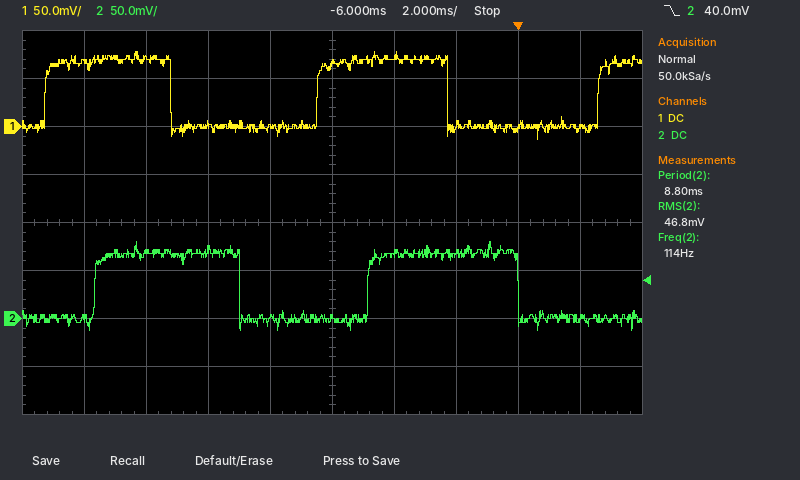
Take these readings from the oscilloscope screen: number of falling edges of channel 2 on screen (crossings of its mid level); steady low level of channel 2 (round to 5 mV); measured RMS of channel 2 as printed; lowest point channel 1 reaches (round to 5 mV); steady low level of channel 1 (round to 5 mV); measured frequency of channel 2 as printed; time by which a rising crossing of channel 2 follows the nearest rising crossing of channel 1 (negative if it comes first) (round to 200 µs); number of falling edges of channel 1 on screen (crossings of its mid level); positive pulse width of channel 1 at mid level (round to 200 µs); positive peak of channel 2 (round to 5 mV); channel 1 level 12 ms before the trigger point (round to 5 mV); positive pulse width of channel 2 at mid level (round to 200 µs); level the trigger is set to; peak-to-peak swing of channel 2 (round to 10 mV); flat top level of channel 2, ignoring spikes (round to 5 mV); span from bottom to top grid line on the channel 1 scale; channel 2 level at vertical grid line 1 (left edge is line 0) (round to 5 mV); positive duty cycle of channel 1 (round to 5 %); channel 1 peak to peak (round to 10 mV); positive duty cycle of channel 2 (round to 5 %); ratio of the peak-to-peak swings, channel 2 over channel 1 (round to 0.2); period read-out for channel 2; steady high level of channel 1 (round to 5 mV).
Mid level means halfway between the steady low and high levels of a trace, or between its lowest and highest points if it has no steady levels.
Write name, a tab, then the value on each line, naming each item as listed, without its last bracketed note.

number of falling edges of channel 2 on screen	2
steady low level of channel 2	0 mV
measured RMS of channel 2 as printed	46.8 mV
lowest point channel 1 reaches	-15 mV
steady low level of channel 1	0 mV
measured frequency of channel 2 as printed	114 Hz
time by which a rising crossing of channel 2 follows the nearest rising crossing of channel 1 (negative if it comes first)	+1.6 ms
number of falling edges of channel 1 on screen	2
positive pulse width of channel 1 at mid level	4.2 ms
positive peak of channel 2	80 mV
channel 1 level 12 ms before the trigger point	70 mV
positive pulse width of channel 2 at mid level	4.8 ms
level the trigger is set to	40.0 mV
peak-to-peak swing of channel 2	90 mV
flat top level of channel 2, ignoring spikes	70 mV
span from bottom to top grid line on the channel 1 scale	400 mV
channel 2 level at vertical grid line 1 (left edge is line 0)	0 mV
positive duty cycle of channel 1	45 %
channel 1 peak to peak	90 mV
positive duty cycle of channel 2	55 %
ratio of the peak-to-peak swings, channel 2 over channel 1	1.0
period read-out for channel 2	8.80 ms
steady high level of channel 1	70 mV
